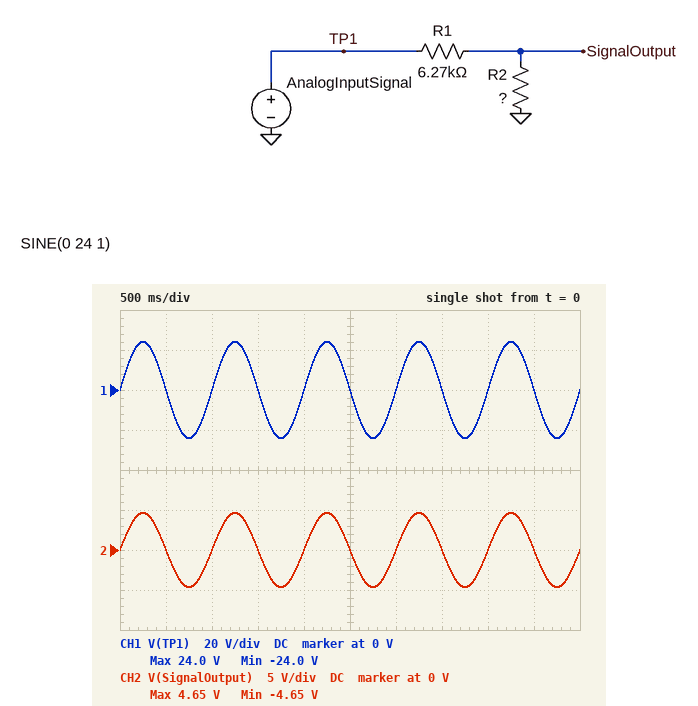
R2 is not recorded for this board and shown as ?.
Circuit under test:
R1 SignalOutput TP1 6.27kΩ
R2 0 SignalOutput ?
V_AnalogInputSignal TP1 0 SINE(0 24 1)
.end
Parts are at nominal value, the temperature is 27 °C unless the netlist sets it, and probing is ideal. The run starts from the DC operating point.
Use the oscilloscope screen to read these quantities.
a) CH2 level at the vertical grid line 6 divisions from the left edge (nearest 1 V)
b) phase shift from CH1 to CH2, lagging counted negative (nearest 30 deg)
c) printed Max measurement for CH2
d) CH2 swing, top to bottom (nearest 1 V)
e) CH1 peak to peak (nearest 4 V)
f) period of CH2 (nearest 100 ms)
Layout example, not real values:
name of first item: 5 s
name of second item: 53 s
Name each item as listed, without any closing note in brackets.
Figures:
CH2 level at the vertical grid line 6 divisions from the left edge: 0 V
phase shift from CH1 to CH2, lagging counted negative: 0 deg
printed Max measurement for CH2: 4.65 V
CH2 swing, top to bottom: 9 V
CH1 peak to peak: 48 V
period of CH2: 1.0 s
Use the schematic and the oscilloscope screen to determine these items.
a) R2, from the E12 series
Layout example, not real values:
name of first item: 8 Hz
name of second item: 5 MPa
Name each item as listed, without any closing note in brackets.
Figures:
R2, from the E12 series: 1.5 kΩ
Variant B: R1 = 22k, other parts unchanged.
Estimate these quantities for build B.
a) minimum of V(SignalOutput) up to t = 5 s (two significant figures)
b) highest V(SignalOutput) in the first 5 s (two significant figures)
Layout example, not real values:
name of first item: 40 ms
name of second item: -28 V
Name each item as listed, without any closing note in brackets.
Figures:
minimum of V(SignalOutput) up to t = 5 s: -1.5 V
highest V(SignalOutput) in the first 5 s: 1.5 V
